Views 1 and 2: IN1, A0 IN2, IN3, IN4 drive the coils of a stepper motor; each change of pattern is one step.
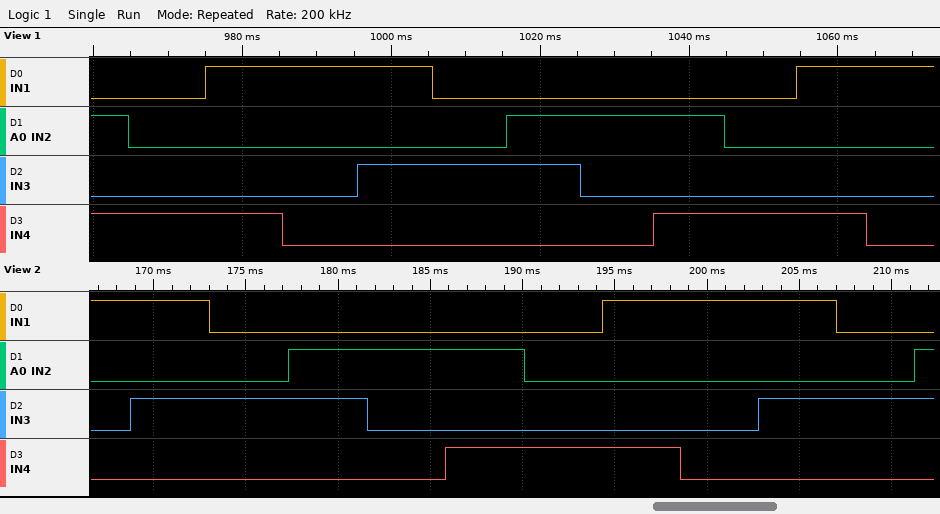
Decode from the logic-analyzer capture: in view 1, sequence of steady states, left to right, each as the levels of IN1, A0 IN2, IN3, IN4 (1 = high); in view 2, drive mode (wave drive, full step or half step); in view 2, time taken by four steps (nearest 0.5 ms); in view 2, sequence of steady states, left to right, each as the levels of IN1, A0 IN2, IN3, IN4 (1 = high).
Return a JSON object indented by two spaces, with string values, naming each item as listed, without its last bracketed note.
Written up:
{
  "in view 1, sequence of steady states, left to right, each as the levels of IN1, A0 IN2, IN3, IN4": "0101 0001 1001 1000 1010 0010 0110 0100 0101 0001 1001 1000",
  "in view 2, drive mode": "half step",
  "in view 2, time taken by four steps": "17.0 ms",
  "in view 2, sequence of steady states, left to right, each as the levels of IN1, A0 IN2, IN3, IN4": "1000 1010 0010 0110 0100 0101 0001 1001 1000 1010 0010 0110"
}
